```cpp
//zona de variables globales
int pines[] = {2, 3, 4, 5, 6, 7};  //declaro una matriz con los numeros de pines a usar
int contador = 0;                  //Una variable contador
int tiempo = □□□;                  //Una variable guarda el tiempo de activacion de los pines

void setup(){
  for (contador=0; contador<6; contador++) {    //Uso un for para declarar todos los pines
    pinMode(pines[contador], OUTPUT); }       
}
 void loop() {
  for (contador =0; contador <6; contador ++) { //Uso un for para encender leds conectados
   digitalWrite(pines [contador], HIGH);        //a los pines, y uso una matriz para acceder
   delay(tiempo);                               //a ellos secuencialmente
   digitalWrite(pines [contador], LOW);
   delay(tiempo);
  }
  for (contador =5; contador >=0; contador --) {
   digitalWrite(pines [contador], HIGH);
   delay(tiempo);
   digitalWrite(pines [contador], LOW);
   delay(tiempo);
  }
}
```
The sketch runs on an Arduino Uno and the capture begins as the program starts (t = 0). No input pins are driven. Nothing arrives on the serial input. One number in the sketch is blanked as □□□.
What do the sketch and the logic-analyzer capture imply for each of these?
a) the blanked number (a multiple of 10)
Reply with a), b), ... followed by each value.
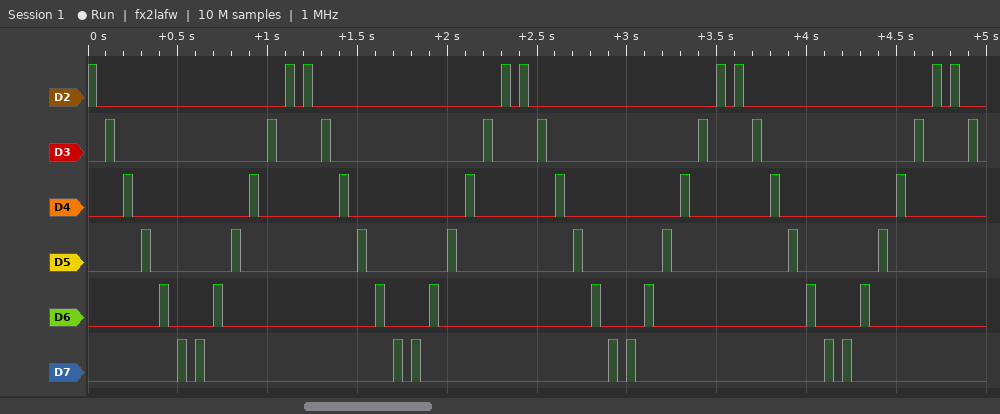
a) 50
